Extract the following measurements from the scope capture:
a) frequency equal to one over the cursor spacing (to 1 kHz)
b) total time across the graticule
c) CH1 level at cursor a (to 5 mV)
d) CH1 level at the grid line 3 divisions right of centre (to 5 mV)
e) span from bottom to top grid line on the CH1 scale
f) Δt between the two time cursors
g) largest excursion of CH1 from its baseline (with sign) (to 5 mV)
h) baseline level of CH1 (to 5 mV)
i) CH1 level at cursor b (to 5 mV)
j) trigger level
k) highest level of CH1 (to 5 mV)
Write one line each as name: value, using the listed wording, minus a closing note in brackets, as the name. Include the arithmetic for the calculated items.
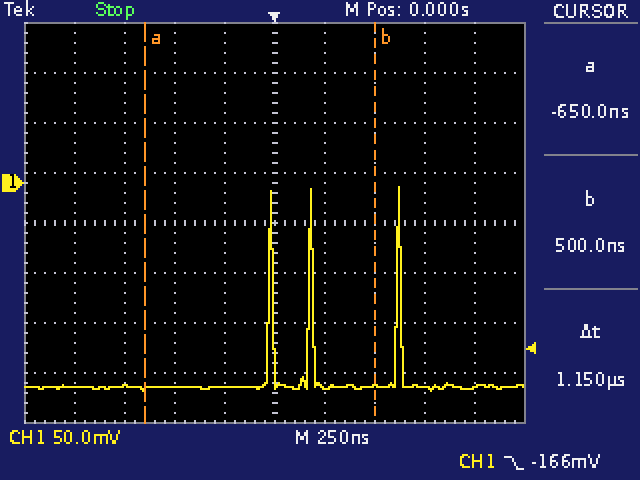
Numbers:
frequency equal to one over the cursor spacing: 1 / 1.15 µs ≈ 870 kHz
total time across the graticule: 2.5 µs
CH1 level at cursor a: -205 mV
CH1 level at the grid line 3 divisions right of centre: -205 mV
span from bottom to top grid line on the CH1 scale: 400 mV
Δt between the two time cursors: 1.15 µs
largest excursion of CH1 from its baseline (with sign): -5 mV − (-205 mV) = +200 mV
baseline level of CH1: -205 mV
CH1 level at cursor b: -205 mV
trigger level: -166 mV
highest level of CH1: -5 mV
